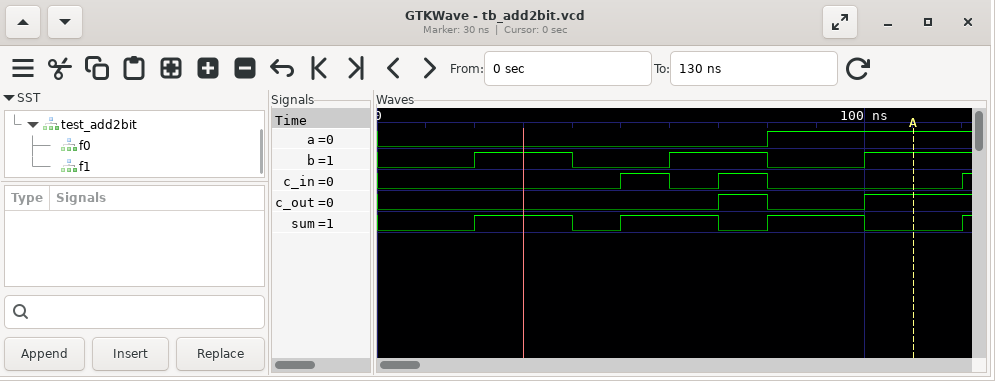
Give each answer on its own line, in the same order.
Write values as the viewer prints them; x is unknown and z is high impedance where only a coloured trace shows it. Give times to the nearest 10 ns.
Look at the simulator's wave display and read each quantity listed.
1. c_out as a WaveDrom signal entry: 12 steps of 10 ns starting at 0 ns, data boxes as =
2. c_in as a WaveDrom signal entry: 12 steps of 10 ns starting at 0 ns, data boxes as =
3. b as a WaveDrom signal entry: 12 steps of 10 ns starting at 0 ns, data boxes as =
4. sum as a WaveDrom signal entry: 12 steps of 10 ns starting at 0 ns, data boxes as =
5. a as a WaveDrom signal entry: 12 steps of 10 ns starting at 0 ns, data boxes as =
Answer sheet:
{name: 'c_out', wave: '0......10.1.'}
{name: 'c_in', wave: '0....1010...'}
{name: 'b', wave: '0.1.0.1.0.1.'}
{name: 'sum', wave: '0.1.01.01.0.'}
{name: 'a', wave: '0.......1...'}
